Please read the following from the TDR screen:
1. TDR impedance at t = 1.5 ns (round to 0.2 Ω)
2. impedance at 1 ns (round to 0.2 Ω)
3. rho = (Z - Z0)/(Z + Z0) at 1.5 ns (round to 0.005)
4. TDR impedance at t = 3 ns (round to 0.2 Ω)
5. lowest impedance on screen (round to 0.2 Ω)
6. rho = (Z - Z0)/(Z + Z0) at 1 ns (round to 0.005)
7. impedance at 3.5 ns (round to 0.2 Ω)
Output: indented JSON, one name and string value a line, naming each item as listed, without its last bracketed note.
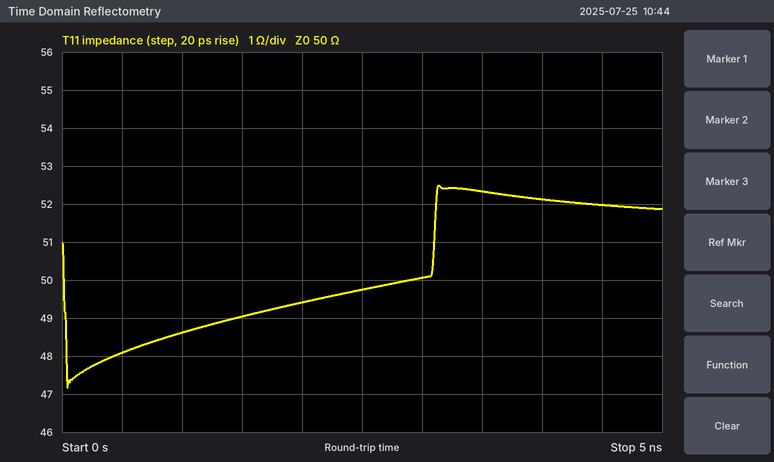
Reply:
{
  "TDR impedance at t = 1.5 ns": "49.0 Ω",
  "impedance at 1 ns": "48.6 Ω",
  "rho = (Z - Z0)/(Z + Z0) at 1.5 ns": "-0.010",
  "TDR impedance at t = 3 ns": "50.0 Ω",
  "lowest impedance on screen": "47.2 Ω",
  "rho = (Z - Z0)/(Z + Z0) at 1 ns": "-0.015",
  "impedance at 3.5 ns": "52.4 Ω"
}
